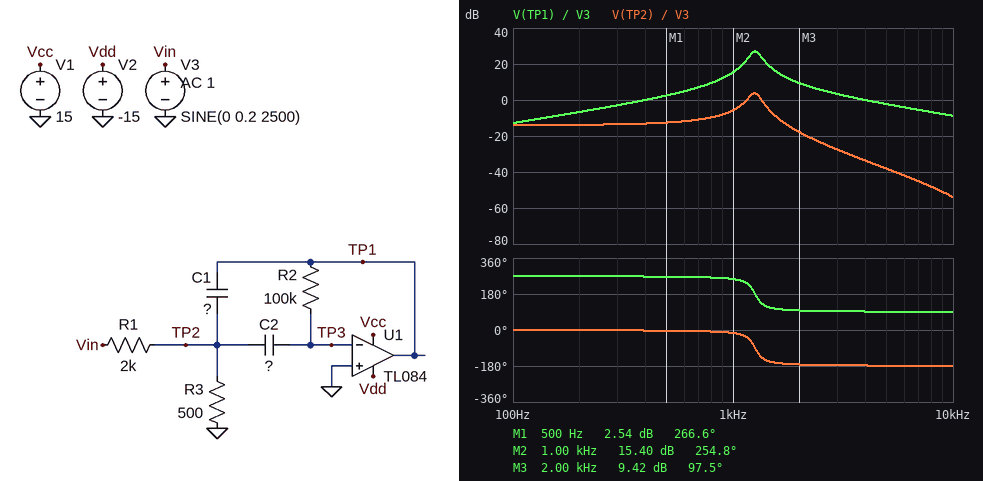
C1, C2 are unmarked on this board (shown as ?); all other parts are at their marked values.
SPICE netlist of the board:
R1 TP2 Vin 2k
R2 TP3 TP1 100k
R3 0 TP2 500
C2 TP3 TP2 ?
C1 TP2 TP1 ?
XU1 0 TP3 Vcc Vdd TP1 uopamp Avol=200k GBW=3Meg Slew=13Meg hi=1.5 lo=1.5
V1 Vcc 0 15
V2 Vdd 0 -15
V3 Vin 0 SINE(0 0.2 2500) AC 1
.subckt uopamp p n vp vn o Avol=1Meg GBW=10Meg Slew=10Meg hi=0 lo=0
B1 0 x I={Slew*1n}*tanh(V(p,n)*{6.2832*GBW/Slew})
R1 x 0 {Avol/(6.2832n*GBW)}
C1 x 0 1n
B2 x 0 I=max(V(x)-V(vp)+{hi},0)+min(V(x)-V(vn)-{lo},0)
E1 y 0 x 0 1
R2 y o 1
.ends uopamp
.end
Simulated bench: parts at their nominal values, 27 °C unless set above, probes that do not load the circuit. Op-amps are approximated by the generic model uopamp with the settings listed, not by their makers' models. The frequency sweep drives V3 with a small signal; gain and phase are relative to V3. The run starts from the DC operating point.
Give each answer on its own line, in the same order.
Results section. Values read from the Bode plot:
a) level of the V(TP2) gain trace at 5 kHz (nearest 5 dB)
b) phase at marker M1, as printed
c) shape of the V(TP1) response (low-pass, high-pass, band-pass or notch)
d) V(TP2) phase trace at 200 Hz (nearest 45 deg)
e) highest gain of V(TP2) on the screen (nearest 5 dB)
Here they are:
-40 dB
266.6 deg
band-pass
0 deg
5 dB
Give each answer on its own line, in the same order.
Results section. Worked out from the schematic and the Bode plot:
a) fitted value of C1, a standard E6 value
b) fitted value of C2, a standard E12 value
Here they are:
22 nF
18 nF
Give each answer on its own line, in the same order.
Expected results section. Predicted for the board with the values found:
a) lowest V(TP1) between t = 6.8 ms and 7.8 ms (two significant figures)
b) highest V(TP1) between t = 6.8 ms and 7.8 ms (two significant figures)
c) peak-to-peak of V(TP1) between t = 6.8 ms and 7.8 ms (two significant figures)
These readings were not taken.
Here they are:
-390 mV
390 mV
780 mV
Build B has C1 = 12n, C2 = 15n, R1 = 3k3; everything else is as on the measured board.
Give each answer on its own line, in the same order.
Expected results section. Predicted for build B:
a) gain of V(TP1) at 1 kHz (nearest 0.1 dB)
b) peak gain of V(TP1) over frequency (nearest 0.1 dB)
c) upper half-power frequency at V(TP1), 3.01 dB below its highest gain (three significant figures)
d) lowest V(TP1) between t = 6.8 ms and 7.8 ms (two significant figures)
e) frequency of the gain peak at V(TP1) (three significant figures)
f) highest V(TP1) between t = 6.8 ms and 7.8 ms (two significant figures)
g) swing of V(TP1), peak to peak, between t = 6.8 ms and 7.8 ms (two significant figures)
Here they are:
5.1 dB
24.5 dB
1.91 kHz
-640 mV
1.79 kHz
640 mV
1.3 V
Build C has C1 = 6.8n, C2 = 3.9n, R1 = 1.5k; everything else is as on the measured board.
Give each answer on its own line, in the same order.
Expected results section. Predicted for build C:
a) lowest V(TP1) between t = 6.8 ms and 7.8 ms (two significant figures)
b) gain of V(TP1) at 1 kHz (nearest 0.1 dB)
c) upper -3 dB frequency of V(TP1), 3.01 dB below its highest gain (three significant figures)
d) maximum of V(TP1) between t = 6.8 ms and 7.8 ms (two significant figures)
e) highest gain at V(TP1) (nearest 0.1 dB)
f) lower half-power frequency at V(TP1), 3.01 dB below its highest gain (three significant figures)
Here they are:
-410 mV
-3.9 dB
5.32 kHz
410 mV
27.7 dB
4.69 kHz
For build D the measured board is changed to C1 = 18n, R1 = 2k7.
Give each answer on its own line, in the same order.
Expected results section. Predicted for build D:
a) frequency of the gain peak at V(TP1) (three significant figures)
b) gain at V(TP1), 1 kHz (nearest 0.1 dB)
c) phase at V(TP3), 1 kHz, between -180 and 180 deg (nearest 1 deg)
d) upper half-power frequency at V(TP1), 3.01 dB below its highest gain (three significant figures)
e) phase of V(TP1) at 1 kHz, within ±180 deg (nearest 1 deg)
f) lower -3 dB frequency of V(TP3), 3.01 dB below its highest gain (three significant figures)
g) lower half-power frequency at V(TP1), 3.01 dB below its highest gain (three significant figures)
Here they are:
1.36 kHz
11.6 dB
167 deg
1.45 kHz
-102 deg
1.28 kHz
1.27 kHz
